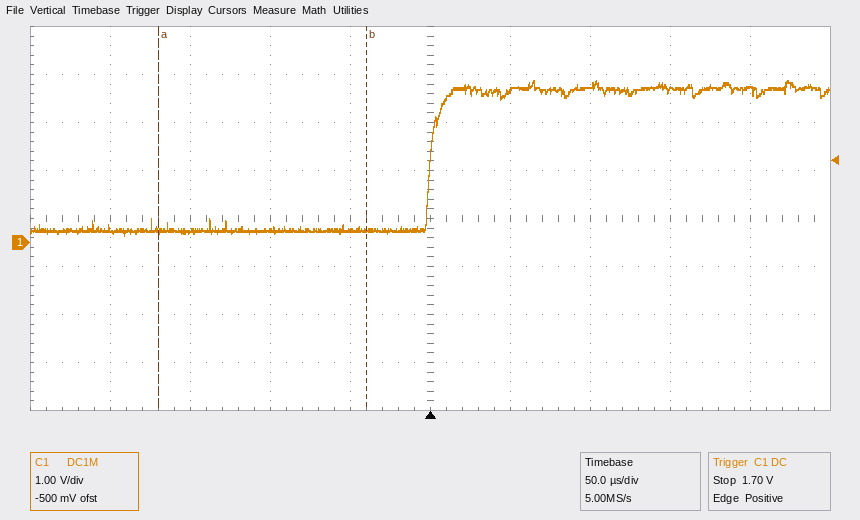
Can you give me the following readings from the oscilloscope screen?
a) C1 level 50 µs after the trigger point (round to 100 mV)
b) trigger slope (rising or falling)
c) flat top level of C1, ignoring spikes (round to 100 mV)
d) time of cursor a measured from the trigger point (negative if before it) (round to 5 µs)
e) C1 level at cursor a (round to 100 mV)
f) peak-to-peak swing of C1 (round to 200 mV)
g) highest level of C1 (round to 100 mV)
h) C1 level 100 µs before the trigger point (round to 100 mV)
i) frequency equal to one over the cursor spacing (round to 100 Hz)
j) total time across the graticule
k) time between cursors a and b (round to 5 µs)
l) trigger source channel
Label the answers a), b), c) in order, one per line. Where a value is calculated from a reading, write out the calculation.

a) 3.2 V
b) rising
c) 3.2 V
d) -170 µs
e) 300 mV
f) 3.2 V
g) 3.4 V
h) 300 mV
i) 1 / 130 µs ≈ 7.7 kHz
j) 500 µs
k) 130 µs
l) C1
